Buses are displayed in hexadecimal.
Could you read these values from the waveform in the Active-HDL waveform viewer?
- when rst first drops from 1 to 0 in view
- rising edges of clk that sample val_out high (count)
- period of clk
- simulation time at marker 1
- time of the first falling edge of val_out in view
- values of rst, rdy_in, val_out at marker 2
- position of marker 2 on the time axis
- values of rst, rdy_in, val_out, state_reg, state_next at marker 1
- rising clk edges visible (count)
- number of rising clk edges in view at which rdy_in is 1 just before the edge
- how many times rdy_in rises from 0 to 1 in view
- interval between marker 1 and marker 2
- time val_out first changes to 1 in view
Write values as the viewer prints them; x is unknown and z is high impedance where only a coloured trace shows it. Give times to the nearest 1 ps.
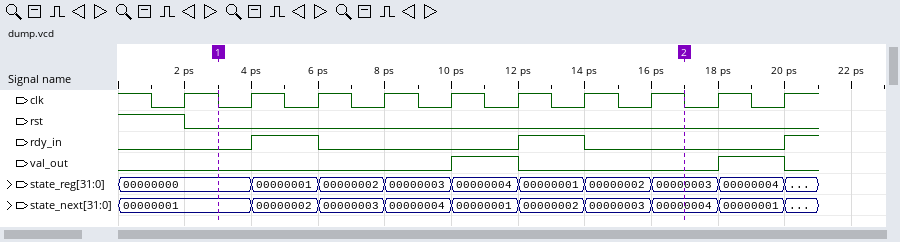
2 ps
2
2 ps
3 ps
12 ps
rst=0, rdy_in=0, val_out=0
17 ps
rst=0, rdy_in=0, val_out=0, state_reg=00000000, state_next=00000001
10
2
3
14 ps
10 ps
